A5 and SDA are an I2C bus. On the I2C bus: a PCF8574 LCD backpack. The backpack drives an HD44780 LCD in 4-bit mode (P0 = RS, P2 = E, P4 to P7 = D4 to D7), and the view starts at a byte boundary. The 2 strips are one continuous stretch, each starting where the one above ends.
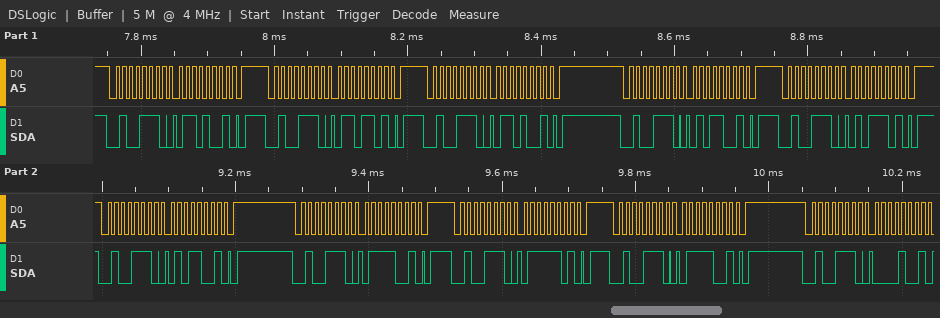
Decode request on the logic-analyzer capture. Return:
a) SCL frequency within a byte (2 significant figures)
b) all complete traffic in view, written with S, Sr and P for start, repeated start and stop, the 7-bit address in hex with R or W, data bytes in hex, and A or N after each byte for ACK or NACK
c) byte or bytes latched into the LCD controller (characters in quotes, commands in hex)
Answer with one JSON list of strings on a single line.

["100 kHz", "S 27W A 69 A P S 27W A 6D A P S 27W A 69 A P S 27W A 59 A P S 27W A 5D A P S 27W A 59 A P S 27W A 79 A P S 27W A 7D A P S 27W A 79 A P S 27W A 09 A", "'e'"]
